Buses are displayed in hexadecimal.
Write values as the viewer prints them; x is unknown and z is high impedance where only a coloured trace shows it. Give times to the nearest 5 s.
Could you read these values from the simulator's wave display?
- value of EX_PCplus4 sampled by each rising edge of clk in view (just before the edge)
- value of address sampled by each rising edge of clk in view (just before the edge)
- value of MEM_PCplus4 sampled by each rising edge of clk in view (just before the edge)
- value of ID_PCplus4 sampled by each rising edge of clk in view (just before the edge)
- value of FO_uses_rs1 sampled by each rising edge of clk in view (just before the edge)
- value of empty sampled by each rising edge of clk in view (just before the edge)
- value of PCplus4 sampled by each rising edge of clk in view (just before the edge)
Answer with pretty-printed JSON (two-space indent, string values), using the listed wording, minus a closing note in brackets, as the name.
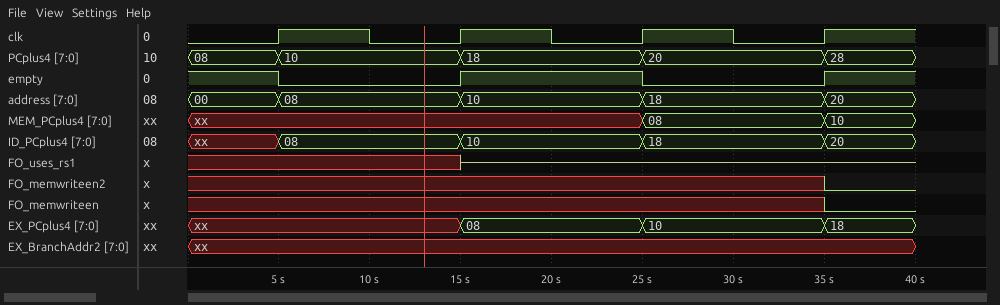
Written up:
{
  "value of EX_PCplus4 sampled by each rising edge of clk in view": "xx, xx, 08, 10",
  "value of address sampled by each rising edge of clk in view": "00, 08, 10, 18",
  "value of MEM_PCplus4 sampled by each rising edge of clk in view": "xx, xx, xx, 08",
  "value of ID_PCplus4 sampled by each rising edge of clk in view": "xx, 08, 10, 18",
  "value of FO_uses_rs1 sampled by each rising edge of clk in view": "x x z z",
  "value of empty sampled by each rising edge of clk in view": "1 0 1 0",
  "value of PCplus4 sampled by each rising edge of clk in view": "08, 10, 18, 20"
}
